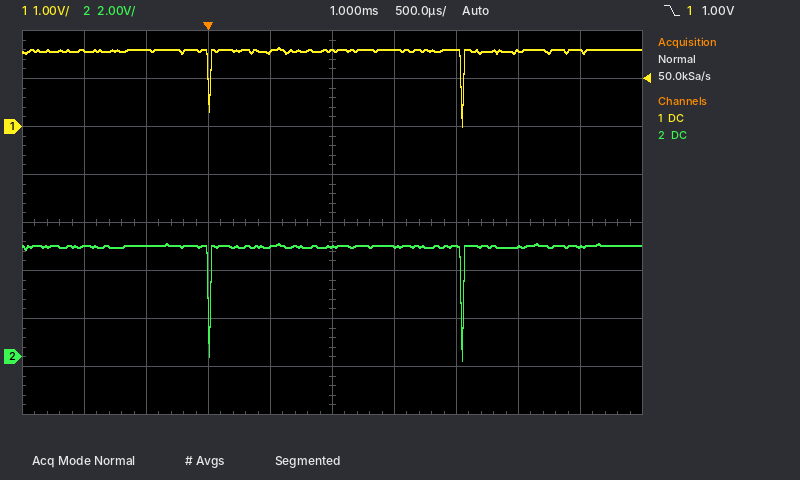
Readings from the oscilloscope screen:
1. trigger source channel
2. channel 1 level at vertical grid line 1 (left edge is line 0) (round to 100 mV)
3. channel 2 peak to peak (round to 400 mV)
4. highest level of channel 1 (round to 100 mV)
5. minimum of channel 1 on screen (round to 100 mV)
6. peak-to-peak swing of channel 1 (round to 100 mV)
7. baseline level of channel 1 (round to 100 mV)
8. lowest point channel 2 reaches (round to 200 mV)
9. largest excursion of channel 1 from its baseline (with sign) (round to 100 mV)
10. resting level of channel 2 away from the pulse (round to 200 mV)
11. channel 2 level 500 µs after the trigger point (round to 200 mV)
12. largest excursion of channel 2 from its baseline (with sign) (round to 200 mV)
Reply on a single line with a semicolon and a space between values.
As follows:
channel 1; 1.6 V; 4.8 V; 1.6 V; 0.0 V; 1.6 V; 1.6 V; -200 mV; -1.6 V; 4.6 V; 4.6 V; -4.8 V
